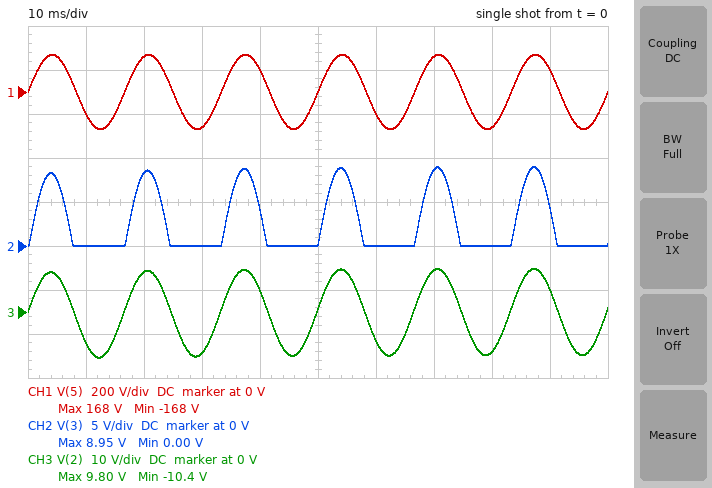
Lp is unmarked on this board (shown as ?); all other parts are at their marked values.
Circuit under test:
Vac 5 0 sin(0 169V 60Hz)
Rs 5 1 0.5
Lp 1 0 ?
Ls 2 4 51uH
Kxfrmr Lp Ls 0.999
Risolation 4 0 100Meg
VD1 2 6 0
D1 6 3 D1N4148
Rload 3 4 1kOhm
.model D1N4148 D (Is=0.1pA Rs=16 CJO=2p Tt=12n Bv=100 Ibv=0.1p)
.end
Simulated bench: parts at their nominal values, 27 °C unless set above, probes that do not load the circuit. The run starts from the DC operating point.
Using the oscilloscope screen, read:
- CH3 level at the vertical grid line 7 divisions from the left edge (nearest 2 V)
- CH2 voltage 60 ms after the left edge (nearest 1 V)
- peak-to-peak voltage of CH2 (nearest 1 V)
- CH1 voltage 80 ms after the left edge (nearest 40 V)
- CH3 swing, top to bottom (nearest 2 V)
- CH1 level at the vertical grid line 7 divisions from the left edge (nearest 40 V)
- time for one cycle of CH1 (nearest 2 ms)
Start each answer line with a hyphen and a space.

- 10 V
- 0 V
- 9 V
- -160 V
- 20 V
- 160 V
- 16 ms
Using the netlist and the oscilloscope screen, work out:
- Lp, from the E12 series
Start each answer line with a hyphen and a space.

- 15 mH
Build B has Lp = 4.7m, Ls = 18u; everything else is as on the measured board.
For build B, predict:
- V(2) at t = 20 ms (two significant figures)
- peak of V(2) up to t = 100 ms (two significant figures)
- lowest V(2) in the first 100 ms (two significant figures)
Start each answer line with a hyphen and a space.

- 9.7 V
- 10 V
- -11 V
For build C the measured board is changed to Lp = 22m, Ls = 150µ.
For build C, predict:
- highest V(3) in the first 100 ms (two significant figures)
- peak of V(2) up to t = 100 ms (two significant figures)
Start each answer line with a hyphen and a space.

- 13 V
- 14 V
